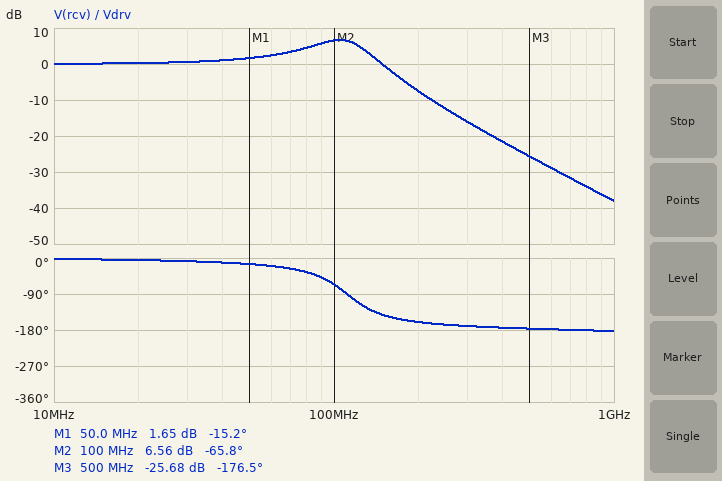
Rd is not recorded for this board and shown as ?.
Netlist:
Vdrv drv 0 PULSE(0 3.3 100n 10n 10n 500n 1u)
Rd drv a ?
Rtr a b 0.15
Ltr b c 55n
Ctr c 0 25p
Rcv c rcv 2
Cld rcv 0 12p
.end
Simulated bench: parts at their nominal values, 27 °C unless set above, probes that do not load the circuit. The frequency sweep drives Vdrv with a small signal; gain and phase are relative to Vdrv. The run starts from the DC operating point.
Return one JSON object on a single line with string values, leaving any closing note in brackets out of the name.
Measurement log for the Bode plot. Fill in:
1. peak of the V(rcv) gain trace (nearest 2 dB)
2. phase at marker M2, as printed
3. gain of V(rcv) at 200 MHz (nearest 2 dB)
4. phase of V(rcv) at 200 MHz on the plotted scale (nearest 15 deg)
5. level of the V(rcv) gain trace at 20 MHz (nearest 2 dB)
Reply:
{"peak of the V(rcv) gain trace": "6 dB", "phase at marker M2, as printed": "-65.8 deg", "gain of V(rcv) at 200 MHz": "-8 dB", "phase of V(rcv) at 200 MHz on the plotted scale": "-165 deg", "level of the V(rcv) gain trace at 20 MHz": "0 dB"}
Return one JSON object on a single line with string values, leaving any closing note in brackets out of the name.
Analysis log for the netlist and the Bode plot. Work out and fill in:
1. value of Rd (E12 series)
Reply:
{"value of Rd": "18 Ω"}
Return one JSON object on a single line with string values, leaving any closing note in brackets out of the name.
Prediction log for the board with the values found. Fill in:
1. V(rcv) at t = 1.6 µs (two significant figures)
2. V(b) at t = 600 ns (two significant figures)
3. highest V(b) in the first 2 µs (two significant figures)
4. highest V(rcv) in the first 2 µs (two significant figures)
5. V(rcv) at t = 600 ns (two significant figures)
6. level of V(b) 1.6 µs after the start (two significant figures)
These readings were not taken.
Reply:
{"V(rcv) at t = 1.6 µs": "3.3 V", "V(b) at t = 600 ns": "3.3 V", "highest V(b) in the first 2 µs": "3.4 V", "highest V(rcv) in the first 2 µs": "3.5 V", "V(rcv) at t = 600 ns": "3.3 V", "level of V(b) 1.6 µs after the start": "3.3 V"}
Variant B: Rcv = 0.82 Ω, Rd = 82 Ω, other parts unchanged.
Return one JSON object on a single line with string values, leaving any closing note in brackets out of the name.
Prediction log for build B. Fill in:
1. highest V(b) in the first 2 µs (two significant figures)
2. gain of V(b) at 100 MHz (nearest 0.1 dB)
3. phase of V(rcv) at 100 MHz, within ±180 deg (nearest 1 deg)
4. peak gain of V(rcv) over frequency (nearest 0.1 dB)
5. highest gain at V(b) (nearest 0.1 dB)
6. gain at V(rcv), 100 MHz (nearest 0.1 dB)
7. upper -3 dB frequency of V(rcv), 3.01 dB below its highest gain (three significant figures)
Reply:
{"highest V(b) in the first 2 µs": "3.3 V", "gain of V(b) at 100 MHz": "-19.8 dB", "phase of V(rcv) at 100 MHz, within ±180 deg": "-84 deg", "peak gain of V(rcv) over frequency": "0 dB", "highest gain at V(b)": "0 dB", "gain at V(rcv), 100 MHz": "-5.7 dB", "upper -3 dB frequency of V(rcv), 3.01 dB below its highest gain": "65.6 MHz"}
